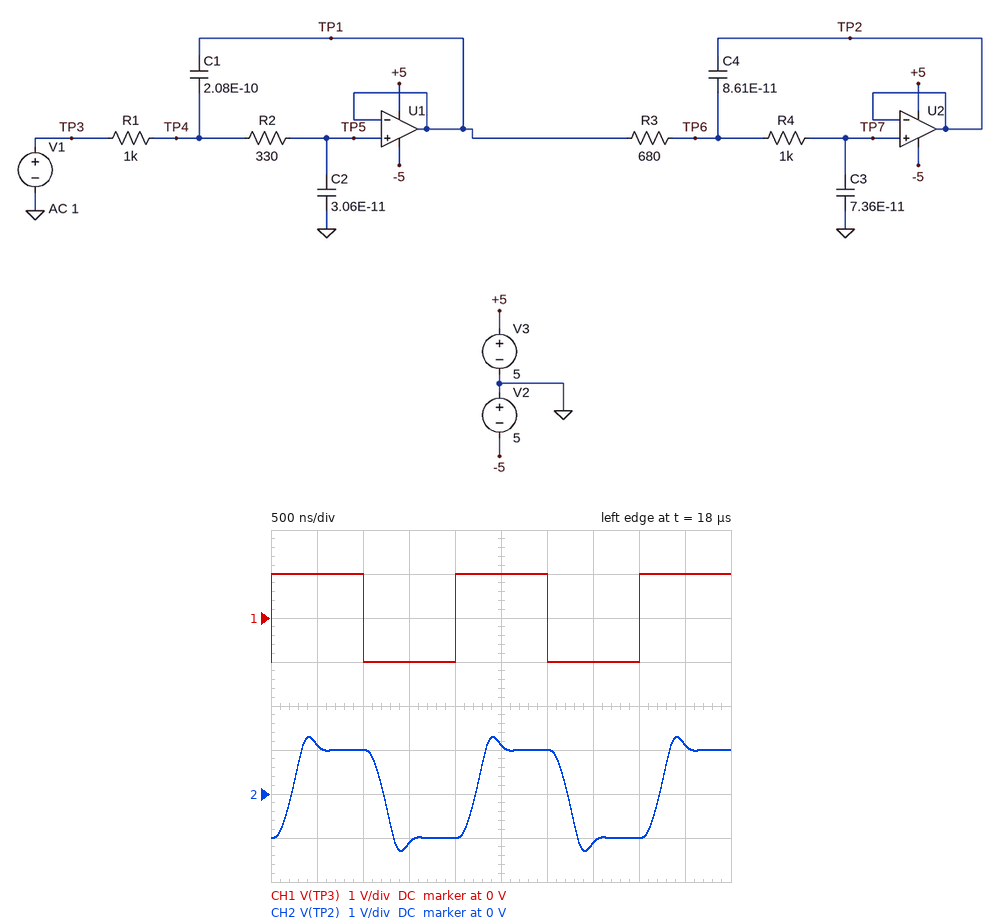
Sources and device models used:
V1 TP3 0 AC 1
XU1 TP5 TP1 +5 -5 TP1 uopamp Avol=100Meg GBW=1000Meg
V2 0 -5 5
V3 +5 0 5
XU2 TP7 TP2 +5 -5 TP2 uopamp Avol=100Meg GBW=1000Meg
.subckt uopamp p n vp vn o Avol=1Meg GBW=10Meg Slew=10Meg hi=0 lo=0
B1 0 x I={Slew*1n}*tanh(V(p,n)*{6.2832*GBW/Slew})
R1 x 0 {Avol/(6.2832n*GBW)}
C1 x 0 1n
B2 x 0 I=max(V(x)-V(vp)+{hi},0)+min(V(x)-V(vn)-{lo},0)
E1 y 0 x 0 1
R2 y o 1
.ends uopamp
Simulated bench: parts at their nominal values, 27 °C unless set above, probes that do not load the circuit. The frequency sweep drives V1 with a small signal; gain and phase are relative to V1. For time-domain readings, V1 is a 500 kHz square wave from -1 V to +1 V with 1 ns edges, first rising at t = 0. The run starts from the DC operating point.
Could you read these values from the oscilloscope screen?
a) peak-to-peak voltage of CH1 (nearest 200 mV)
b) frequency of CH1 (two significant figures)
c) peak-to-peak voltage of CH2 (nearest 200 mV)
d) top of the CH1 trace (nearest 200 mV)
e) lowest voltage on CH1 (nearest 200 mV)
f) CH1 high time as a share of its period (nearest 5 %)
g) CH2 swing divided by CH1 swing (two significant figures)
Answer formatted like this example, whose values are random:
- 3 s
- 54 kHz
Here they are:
- 2.0 V
- 500 kHz
- 2.6 V
- 1.0 V
- -1.0 V
- 50 %
- 1.3
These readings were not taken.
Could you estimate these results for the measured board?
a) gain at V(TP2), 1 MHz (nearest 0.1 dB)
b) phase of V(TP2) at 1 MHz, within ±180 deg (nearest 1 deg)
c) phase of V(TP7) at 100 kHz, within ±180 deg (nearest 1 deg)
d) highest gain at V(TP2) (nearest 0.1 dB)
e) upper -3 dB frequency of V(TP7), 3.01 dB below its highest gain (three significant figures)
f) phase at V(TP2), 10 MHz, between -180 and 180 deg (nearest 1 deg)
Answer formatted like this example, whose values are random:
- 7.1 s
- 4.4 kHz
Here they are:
- -0.7 dB
- -59 deg
- -6 deg
- 0 dB
- 2.23 MHz
- 44 deg
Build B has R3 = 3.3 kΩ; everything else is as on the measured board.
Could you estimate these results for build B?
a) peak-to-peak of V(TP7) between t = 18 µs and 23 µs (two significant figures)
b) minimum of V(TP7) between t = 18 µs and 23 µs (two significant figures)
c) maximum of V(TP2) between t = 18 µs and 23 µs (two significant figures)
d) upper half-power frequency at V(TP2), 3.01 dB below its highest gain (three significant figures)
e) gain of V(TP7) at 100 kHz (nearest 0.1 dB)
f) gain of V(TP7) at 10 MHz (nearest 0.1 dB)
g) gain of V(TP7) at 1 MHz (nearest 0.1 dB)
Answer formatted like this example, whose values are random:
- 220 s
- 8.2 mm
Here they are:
- 1.9 V
- -960 mV
- 960 mV
- 648 kHz
- -0.1 dB
- -56.4 dB
- -5.6 dB
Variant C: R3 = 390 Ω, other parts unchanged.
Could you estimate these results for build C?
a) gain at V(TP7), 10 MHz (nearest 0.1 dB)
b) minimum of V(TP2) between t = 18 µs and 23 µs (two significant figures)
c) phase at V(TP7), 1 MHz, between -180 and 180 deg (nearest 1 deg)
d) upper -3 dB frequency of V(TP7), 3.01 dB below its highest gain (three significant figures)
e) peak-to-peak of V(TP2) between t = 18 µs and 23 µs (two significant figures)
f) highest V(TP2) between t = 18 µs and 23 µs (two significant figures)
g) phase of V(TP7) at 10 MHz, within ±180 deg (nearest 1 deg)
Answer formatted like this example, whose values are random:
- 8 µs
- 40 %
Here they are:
- -38.6 dB
- -1.4 V
- -51 deg
- 2.75 MHz
- 2.7 V
- 1.4 V
- 55 deg
